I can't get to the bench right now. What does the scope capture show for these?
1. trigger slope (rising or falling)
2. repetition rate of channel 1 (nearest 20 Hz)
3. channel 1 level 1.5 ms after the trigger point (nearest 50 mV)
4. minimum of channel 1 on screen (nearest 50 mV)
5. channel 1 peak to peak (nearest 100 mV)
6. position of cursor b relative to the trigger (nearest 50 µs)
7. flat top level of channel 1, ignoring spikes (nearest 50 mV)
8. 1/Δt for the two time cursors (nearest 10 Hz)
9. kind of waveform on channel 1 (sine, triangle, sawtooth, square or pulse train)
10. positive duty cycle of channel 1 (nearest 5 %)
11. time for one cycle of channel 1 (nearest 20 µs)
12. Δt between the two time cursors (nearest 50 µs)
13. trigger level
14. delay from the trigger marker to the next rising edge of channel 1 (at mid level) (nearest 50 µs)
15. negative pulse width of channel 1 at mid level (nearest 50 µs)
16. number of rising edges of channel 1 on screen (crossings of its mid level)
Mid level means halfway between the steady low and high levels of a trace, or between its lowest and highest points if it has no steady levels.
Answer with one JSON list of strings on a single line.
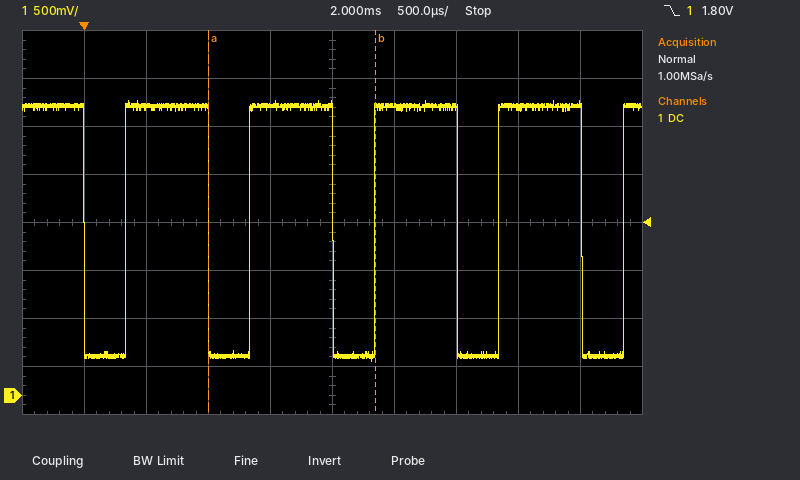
["falling", "1.00 kHz", "3.00 V", "350 mV", "2.70 V", "+2.35 ms", "3.00 V", "740 Hz", "pulse train", "65 %", "1.00 ms", "1.35 ms", "1.80 V", "350 µs", "350 µs", "5"]
